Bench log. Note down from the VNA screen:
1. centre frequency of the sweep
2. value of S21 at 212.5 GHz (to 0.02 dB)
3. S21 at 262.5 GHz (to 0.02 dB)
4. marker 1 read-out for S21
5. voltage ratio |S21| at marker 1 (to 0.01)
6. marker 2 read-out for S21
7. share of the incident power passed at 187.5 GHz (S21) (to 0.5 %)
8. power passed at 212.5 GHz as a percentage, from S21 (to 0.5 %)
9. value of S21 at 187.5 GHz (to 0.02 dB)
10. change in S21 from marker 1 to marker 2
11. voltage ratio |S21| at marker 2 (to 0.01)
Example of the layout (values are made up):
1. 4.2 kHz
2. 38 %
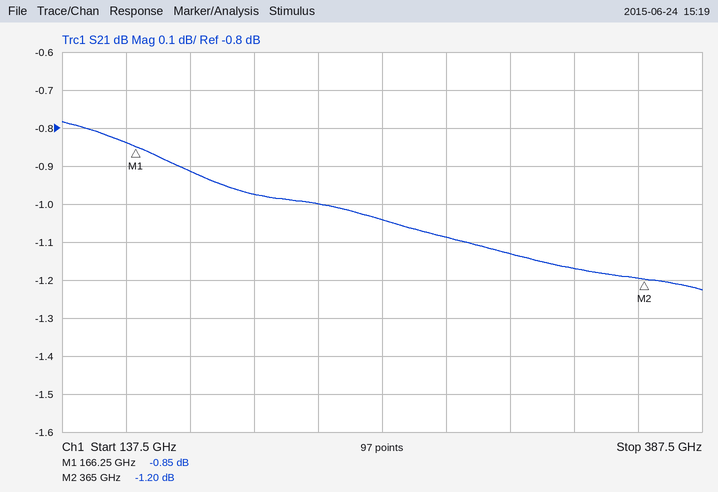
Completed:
1. 262.5 GHz
2. -0.98 dB
3. -1.04 dB
4. -0.85 dB
5. 0.91
6. -1.20 dB
7. 81.0 %
8. 80.0 %
9. -0.92 dB
10. -0.35 dB
11. 0.87
